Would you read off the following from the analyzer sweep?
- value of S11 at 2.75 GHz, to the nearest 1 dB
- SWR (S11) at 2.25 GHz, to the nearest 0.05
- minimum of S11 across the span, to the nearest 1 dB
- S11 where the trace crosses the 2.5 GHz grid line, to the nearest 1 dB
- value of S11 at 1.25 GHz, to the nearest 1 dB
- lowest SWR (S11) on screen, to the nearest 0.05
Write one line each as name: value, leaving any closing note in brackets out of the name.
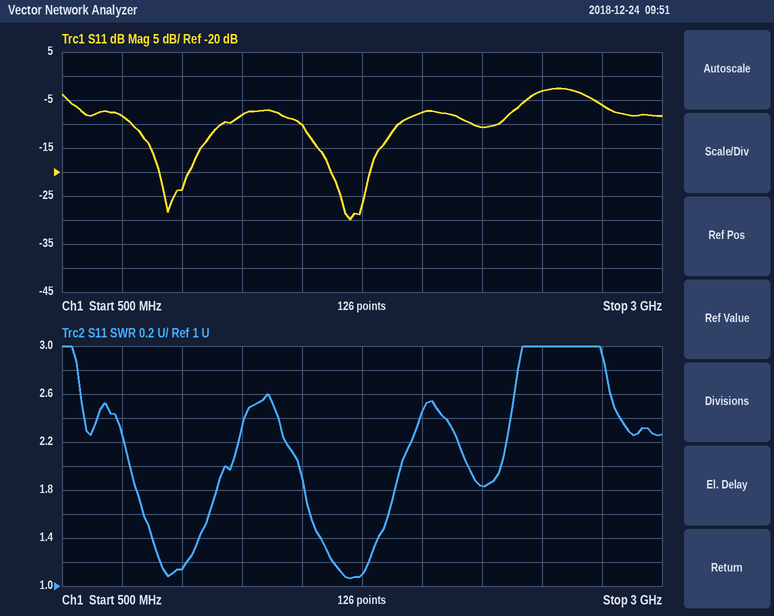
value of S11 at 2.75 GHz, to the nearest 1 dB: -6 dB
SWR (S11) at 2.25 GHz, to the nearest 0.05: 1.85
minimum of S11 across the span, to the nearest 1 dB: -30 dB
S11 where the trace crosses the 2.5 GHz grid line, to the nearest 1 dB: -3 dB
value of S11 at 1.25 GHz, to the nearest 1 dB: -8 dB
lowest SWR (S11) on screen, to the nearest 0.05: 1.05
